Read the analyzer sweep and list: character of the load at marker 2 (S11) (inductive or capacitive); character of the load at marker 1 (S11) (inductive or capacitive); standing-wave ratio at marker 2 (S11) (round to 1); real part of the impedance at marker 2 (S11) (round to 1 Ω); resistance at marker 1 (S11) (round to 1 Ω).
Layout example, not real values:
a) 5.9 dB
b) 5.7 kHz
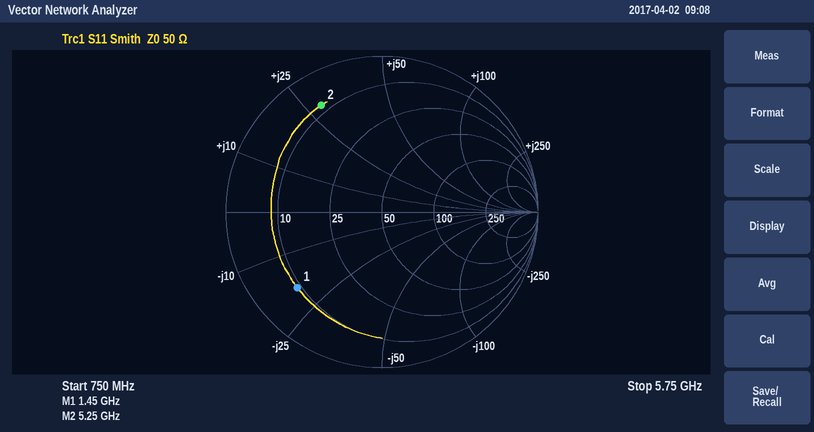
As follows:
a) inductive
b) capacitive
c) 8
d) 8 Ω
e) 9 Ω
